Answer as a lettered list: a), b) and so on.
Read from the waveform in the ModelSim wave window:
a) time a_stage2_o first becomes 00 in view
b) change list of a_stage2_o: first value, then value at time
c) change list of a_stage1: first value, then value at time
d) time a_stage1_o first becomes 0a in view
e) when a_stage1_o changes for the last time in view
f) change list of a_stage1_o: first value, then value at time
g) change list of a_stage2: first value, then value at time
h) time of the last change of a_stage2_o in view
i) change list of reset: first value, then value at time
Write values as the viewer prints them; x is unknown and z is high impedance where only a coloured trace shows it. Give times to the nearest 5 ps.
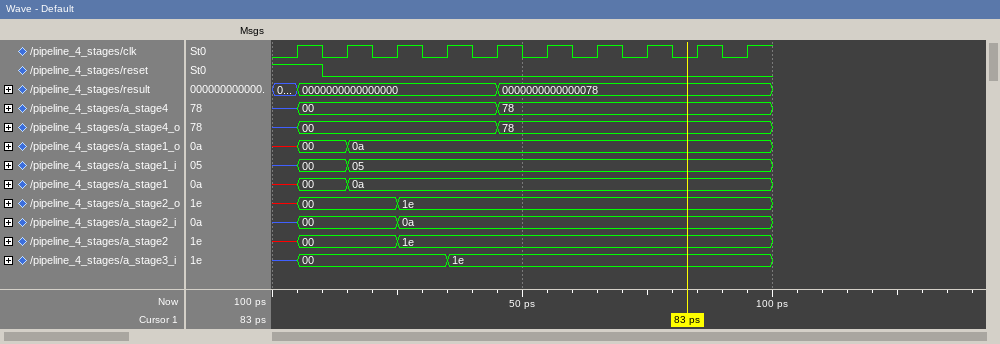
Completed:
a) 5 ps
b) x, 00 at 5 ps, 1e at 25 ps
c) x, 00 at 5 ps, 0a at 15 ps
d) 15 ps
e) 15 ps
f) x, 00 at 5 ps, 0a at 15 ps
g) x, 00 at 5 ps, 1e at 25 ps
h) 25 ps
i) 1, 0 at 10 ps
